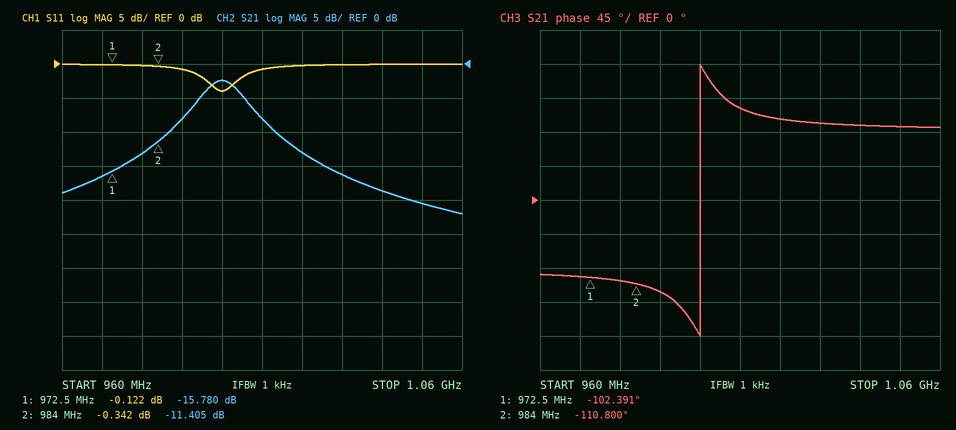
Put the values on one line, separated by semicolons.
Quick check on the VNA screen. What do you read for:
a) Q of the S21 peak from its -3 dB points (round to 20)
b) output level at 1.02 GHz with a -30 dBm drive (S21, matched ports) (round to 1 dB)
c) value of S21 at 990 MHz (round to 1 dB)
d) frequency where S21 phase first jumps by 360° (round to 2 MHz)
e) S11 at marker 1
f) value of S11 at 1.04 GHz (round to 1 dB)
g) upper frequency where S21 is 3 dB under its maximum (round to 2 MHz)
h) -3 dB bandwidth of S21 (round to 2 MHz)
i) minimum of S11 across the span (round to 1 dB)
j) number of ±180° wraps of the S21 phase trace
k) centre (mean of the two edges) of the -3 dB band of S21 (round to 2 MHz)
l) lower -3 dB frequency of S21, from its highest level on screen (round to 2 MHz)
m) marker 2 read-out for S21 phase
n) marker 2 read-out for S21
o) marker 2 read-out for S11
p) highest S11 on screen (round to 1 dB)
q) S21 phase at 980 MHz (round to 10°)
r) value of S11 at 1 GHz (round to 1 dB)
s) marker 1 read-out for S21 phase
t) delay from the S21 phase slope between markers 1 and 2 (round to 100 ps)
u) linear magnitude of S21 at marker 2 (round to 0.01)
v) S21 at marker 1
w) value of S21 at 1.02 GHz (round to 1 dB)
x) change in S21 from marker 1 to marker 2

80; -43 dBm; -8 dB; 1.000 GHz; -0.122 dB; 0 dB; 1.006 GHz; 12 MHz; -4 dB; 1; 1.000 GHz; 994 MHz; -110.800°; -11.405 dB; -0.342 dB; 0 dB; -110°; -4 dB; -102.391°; 2.0 ns; 0.27; -15.780 dB; -13 dB; 4.375 dB
